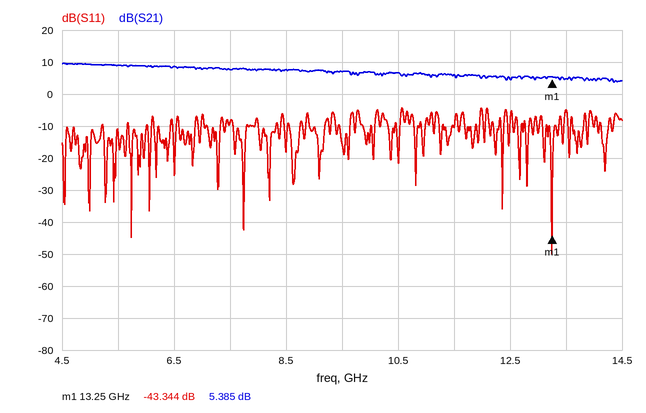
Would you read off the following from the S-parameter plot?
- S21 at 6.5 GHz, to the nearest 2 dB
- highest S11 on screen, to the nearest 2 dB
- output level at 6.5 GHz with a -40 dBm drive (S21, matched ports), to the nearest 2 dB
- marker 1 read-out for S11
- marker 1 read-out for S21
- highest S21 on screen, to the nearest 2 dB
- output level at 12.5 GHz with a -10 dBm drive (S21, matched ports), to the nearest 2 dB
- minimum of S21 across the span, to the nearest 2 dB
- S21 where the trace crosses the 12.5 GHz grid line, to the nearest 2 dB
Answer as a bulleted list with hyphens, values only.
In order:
- 8 dB
- -4 dB
- -32 dBm
- -43.344 dB
- 5.385 dB
- 10 dB
- -6 dBm
- 4 dB
- 4 dB
